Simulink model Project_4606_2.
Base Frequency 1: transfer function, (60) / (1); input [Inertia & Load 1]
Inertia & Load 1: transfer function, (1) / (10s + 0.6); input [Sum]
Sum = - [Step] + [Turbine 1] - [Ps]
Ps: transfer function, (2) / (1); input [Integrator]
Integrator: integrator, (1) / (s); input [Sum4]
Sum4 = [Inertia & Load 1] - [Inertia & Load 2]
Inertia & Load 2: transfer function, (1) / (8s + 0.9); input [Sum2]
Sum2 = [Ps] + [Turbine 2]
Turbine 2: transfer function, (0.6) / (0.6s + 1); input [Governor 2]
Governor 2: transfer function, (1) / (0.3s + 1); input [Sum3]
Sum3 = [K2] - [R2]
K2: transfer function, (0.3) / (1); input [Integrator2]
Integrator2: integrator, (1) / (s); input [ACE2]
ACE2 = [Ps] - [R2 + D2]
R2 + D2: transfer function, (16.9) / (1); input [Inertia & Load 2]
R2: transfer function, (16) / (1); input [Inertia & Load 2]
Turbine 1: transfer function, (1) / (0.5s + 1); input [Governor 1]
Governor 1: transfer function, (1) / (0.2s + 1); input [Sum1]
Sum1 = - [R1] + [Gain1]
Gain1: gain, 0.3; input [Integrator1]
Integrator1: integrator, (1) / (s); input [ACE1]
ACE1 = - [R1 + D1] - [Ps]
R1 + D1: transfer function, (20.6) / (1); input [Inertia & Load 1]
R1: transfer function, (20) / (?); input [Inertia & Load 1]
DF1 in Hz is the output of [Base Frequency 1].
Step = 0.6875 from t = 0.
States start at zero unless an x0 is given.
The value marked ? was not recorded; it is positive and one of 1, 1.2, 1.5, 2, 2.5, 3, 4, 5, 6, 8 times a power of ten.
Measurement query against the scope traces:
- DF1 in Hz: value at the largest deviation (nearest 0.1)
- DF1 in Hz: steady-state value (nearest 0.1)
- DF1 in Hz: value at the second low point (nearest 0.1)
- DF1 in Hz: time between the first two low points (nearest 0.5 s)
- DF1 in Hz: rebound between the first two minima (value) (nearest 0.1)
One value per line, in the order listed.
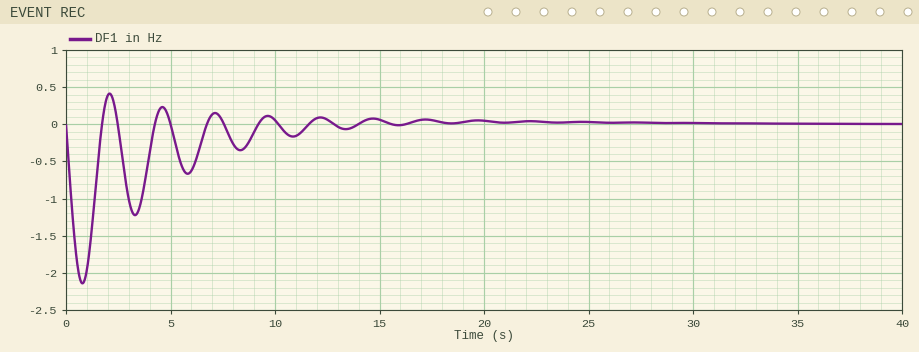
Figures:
-2.1
0.0
-1.2
2.5 s
0.4
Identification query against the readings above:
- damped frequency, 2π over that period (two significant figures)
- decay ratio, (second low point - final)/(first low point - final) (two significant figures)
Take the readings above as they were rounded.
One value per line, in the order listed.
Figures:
2.5 rad/s
0.57
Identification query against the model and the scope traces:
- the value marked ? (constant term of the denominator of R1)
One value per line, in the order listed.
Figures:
0.5
